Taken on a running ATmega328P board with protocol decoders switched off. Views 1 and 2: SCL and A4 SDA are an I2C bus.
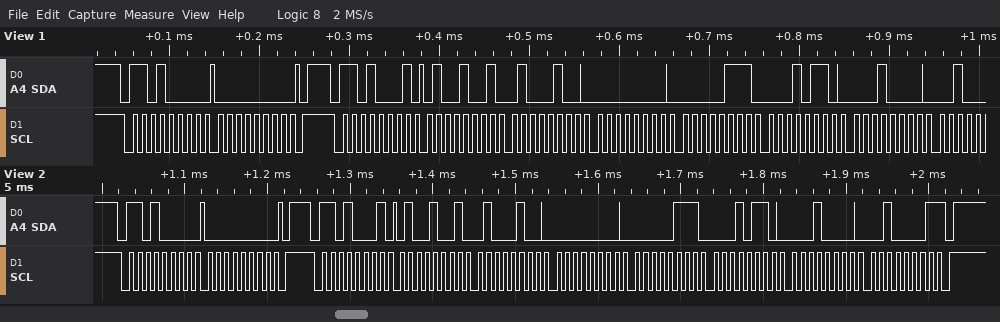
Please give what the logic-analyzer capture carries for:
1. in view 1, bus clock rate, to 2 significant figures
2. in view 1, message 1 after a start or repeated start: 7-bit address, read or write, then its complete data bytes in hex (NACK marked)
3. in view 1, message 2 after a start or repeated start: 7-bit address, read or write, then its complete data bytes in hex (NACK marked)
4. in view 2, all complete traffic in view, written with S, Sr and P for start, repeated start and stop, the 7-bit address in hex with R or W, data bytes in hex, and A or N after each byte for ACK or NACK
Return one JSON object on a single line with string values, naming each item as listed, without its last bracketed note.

{"in view 1, bus clock rate, to 2 significant figures": "100 kHz", "in view 1, message 1 after a start or repeated start: 7-bit address, read or write, then its complete data bytes in hex": "0x68 write: 00", "in view 1, message 2 after a start or repeated start: 7-bit address, read or write, then its complete data bytes in hex": "0x68 read: 49 44 00 07 16 10", "in view 2, all complete traffic in view, written with S, Sr and P for start, repeated start and stop, the 7-bit address in hex with R or W, data bytes in hex, and A or N after each byte for ACK or NACK": "S 68W A 00 A P S 68R A 49 A 44 A 00 A 07 A 16 A 10 A 21 N P"}
